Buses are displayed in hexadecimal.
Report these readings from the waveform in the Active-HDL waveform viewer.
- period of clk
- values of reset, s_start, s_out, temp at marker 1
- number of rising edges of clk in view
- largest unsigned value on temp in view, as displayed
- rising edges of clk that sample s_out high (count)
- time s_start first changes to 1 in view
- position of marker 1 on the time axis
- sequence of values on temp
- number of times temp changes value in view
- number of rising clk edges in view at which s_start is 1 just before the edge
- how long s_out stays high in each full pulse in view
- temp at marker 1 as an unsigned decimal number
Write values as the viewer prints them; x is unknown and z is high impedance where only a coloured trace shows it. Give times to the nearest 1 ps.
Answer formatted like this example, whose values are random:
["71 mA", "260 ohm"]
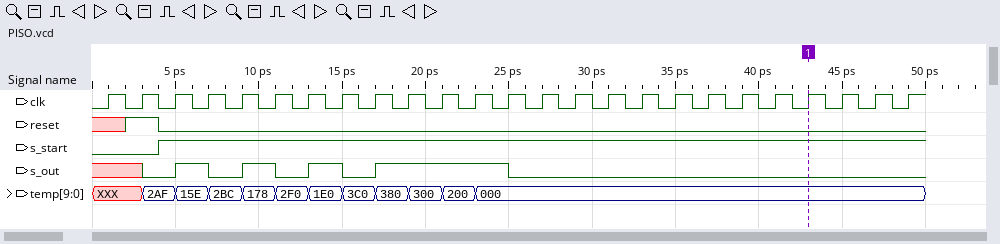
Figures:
["2 ps", "reset=0, s_start=1, s_out=0, temp=000", "25", "3C0", "7", "4 ps", "43 ps", "XXX, 2AF, 15E, 2BC, 178, 2F0, 1E0, 3C0, 380, 300, 200, 000", "11", "23", "2 ps, 2 ps, 2 ps, 8 ps", "0"]
